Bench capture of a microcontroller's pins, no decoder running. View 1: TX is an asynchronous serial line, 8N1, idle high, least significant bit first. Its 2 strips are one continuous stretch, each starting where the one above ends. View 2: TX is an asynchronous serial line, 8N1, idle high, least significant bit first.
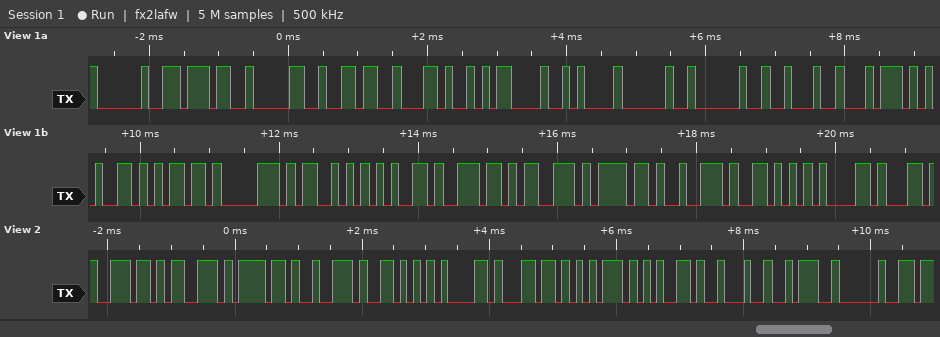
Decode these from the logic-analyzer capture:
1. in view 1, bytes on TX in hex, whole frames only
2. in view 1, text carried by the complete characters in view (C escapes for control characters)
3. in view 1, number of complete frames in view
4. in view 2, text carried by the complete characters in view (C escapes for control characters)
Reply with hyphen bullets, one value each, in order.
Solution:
- 20 37 30 36 2C 0D 0A 20 20 22 74 65 6D 70 53 65 6E 73 6F 72 56 61
- " 706,\r\n  \"tempSensorVa"
- 22
- "nsorValue\": "
